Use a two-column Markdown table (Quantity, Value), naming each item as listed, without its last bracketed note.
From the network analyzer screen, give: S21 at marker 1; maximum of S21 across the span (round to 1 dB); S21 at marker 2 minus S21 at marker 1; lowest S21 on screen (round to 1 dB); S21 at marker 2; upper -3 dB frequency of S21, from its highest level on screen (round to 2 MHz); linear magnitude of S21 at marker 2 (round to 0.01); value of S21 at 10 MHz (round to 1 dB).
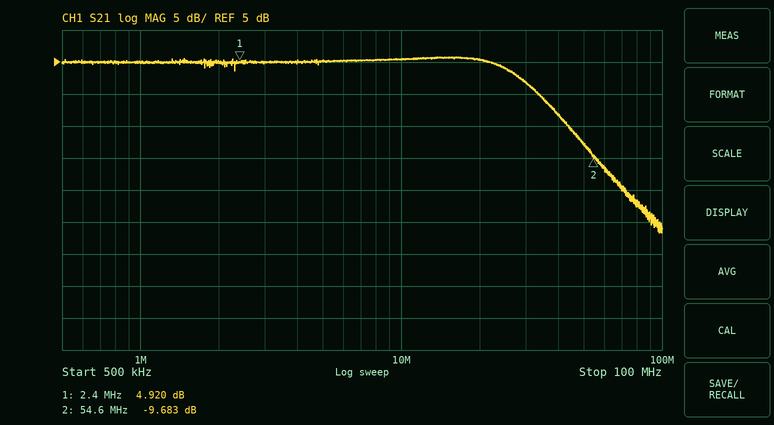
| Quantity | Value |
|---|---|
| S21 at marker 1 | 4.920 dB |
| maximum of S21 across the span | 6 dB |
| S21 at marker 2 minus S21 at marker 1 | -14.603 dB |
| lowest S21 on screen | -22 dB |
| S21 at marker 2 | -9.683 dB |
| upper -3 dB frequency of S21, from its highest level on screen | 28 MHz |
| linear magnitude of S21 at marker 2 | 0.33 |
| value of S21 at 10 MHz | 5 dB |
